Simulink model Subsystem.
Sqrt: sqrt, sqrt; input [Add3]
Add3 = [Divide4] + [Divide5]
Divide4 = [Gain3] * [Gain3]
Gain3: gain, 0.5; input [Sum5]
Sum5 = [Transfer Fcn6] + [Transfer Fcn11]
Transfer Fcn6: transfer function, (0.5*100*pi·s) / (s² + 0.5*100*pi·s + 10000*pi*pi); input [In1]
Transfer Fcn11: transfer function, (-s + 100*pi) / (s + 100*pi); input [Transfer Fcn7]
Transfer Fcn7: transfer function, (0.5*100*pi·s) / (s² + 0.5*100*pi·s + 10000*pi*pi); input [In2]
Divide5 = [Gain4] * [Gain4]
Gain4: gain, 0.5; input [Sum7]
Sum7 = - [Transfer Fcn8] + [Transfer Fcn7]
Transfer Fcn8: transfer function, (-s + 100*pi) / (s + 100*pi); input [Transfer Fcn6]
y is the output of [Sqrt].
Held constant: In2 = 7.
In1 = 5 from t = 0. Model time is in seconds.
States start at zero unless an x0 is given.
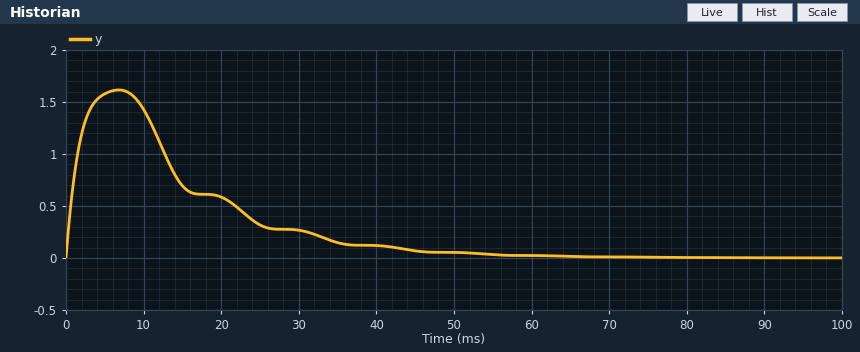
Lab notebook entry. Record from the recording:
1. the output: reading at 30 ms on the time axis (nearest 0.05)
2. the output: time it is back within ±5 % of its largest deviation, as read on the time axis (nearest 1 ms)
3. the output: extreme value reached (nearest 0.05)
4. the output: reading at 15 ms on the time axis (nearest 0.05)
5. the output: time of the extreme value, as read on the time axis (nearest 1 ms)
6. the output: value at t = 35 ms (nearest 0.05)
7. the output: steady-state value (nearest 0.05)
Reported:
0.25
44 ms
1.60
0.70
7 ms
0.15
0.00
